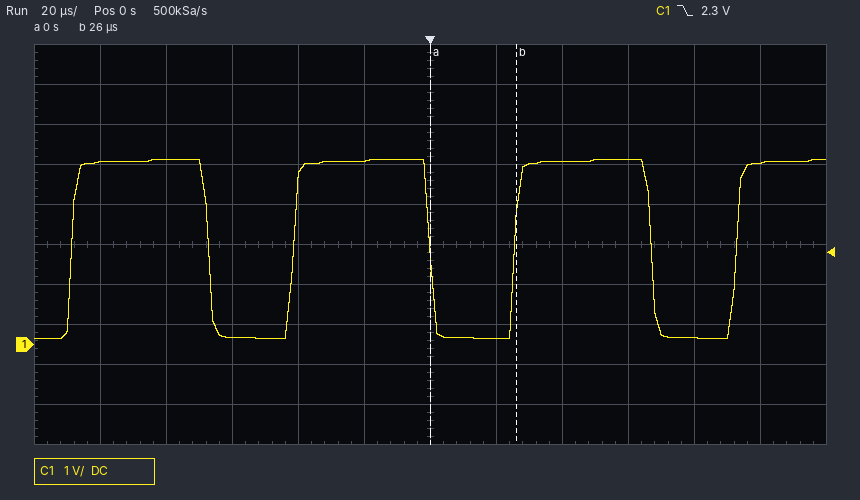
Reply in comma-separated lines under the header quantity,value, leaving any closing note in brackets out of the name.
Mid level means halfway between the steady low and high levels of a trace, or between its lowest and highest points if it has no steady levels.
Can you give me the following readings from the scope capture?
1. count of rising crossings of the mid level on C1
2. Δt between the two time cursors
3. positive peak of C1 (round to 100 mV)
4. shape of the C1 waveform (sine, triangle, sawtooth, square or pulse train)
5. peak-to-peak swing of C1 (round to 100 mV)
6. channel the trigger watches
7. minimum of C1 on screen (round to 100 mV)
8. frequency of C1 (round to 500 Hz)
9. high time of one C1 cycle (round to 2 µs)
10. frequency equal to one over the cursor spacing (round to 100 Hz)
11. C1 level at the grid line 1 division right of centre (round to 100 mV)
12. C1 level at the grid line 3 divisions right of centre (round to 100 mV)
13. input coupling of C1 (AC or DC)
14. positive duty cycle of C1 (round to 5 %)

quantity,value
count of rising crossings of the mid level on C1,4
Δt between the two time cursors,26 µs
positive peak of C1,4.6 V
shape of the C1 waveform,pulse train
peak-to-peak swing of C1,4.5 V
channel the trigger watches,C1
minimum of C1 on screen,100 mV
frequency of C1,15.0 kHz
high time of one C1 cycle,42 µs
frequency equal to one over the cursor spacing,38.5 kHz
C1 level at the grid line 1 division right of centre,100 mV
C1 level at the grid line 3 divisions right of centre,4.6 V
input coupling of C1,DC
positive duty cycle of C1,60 %
